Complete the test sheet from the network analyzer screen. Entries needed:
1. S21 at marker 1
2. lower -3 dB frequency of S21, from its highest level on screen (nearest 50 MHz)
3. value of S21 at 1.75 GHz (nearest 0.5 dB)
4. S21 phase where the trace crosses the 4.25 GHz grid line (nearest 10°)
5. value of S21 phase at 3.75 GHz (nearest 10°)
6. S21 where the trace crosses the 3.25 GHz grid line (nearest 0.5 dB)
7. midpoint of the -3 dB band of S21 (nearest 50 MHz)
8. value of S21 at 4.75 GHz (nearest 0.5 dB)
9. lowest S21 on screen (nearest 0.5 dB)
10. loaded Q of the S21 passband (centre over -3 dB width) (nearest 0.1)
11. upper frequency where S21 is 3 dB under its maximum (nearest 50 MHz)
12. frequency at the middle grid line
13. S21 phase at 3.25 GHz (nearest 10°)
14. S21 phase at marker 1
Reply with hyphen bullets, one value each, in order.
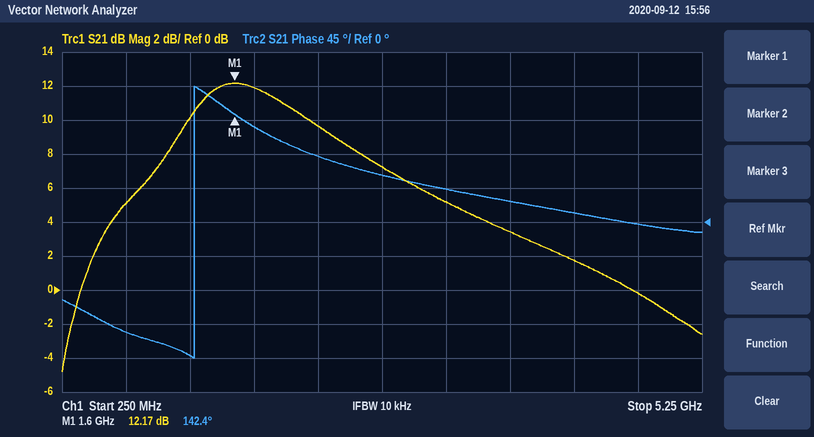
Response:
- 12.17 dB
- 1.15 GHz
- 12.0 dB
- 10°
- 30°
- 5.0 dB
- 1.75 GHz
- 0.0 dB
- -5.0 dB
- 1.5
- 2.35 GHz
- 2.75 GHz
- 40°
- 142.4°
